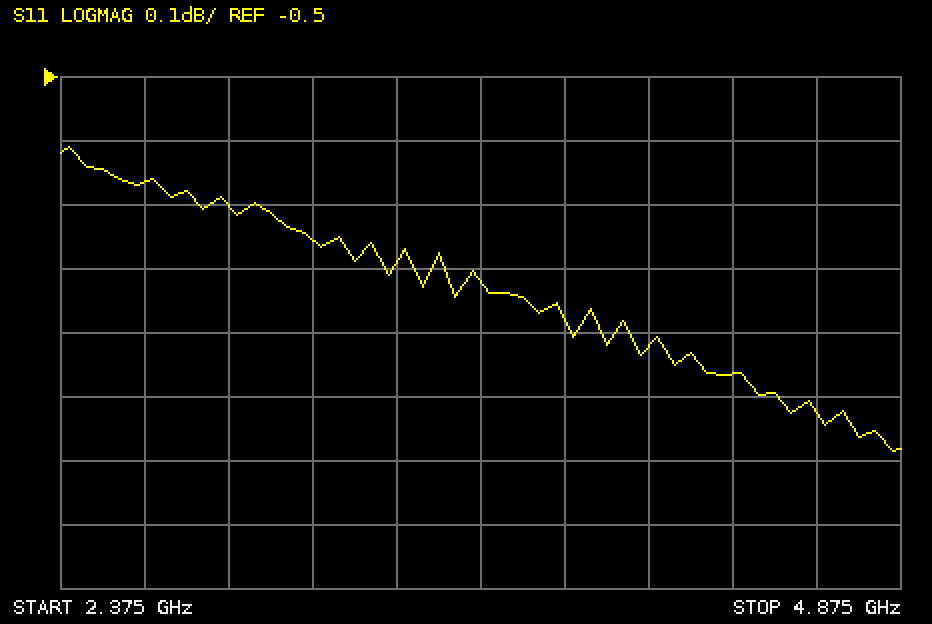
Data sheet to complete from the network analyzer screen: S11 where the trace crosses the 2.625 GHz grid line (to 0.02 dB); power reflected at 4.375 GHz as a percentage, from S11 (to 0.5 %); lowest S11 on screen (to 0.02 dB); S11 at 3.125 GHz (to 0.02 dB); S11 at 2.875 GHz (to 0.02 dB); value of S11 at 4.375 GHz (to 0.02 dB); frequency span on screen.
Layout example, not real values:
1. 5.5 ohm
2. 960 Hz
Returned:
1. -0.66 dB
2. 80.0 %
3. -1.08 dB
4. -0.76 dB
5. -0.70 dB
6. -0.96 dB
7. 2.5 GHz
